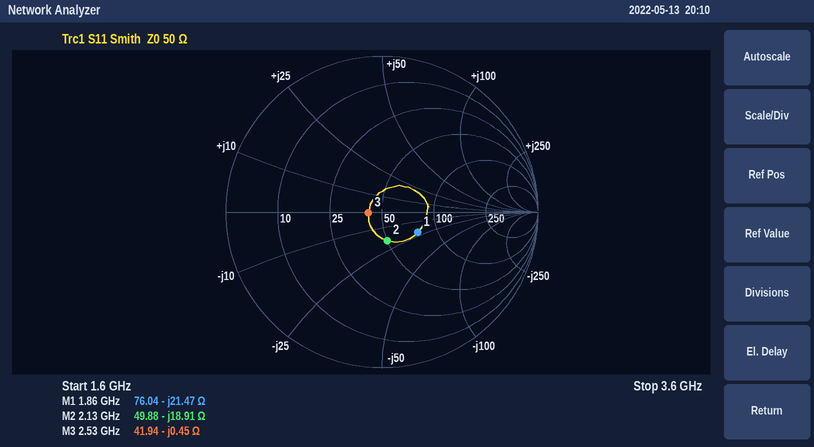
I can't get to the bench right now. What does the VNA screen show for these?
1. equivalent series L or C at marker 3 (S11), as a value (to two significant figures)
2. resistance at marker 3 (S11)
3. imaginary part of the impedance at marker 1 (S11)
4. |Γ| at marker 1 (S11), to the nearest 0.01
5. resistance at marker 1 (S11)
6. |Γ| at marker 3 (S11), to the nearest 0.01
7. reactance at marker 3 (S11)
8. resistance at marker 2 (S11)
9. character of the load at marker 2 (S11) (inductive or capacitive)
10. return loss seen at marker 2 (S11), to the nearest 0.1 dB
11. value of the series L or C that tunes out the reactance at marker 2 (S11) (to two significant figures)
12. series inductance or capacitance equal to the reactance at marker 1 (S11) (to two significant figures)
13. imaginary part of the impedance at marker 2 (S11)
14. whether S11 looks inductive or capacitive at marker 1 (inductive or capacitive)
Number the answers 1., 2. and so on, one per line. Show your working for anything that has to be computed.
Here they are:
1. C = 1/(2π × 2.53 GHz × 0.45 Ω) ≈ 140 pF
2. 41.94 Ω
3. -21.47 Ω
4. 0.26
5. 76.04 Ω
6. 0.09
7. -0.45 Ω
8. 49.88 Ω
9. capacitive
10. 14.6 dB
11. L = 18.91 Ω/(2π × 2.13 GHz) ≈ 1.4 nH
12. C = 1/(2π × 1.86 GHz × 21.47 Ω) ≈ 4.0 pF
13. -18.91 Ω
14. capacitive
